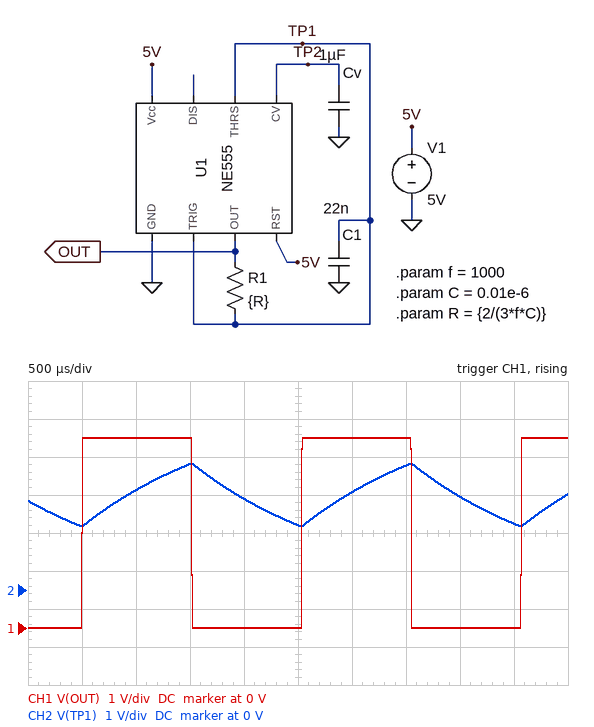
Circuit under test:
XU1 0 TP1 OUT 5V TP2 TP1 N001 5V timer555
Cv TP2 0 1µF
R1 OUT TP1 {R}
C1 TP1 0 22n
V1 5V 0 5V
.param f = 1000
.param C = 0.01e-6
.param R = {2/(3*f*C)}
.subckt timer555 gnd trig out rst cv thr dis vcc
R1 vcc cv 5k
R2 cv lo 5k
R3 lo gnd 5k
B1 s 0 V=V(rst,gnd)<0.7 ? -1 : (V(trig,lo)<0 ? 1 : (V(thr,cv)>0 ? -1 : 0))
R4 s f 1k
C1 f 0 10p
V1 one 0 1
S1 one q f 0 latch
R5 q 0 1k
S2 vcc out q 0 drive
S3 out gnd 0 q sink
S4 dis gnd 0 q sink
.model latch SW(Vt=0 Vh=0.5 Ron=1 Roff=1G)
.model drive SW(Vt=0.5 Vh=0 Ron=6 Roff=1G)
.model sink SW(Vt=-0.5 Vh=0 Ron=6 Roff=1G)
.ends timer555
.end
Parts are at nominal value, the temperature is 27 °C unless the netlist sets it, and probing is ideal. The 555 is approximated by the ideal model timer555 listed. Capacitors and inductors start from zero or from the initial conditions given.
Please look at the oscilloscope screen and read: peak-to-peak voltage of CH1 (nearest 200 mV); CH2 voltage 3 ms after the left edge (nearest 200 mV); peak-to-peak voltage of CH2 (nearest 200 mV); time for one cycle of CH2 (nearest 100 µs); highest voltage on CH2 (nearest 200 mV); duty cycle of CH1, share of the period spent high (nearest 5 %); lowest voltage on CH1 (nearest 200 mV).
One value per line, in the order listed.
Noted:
5.0 V
2.6 V
1.6 V
2.0 ms
3.4 V
50 %
0 V
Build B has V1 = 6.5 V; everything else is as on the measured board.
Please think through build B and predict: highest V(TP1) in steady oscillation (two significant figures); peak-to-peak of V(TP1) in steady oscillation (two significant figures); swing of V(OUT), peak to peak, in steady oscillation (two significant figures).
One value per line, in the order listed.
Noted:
4.3 V
2.2 V
6.5 V
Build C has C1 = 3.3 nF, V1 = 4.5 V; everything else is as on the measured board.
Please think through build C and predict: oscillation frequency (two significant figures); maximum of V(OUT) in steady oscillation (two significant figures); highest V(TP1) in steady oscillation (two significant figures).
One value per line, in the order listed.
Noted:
3.3 kHz
4.5 V
3.0 V
